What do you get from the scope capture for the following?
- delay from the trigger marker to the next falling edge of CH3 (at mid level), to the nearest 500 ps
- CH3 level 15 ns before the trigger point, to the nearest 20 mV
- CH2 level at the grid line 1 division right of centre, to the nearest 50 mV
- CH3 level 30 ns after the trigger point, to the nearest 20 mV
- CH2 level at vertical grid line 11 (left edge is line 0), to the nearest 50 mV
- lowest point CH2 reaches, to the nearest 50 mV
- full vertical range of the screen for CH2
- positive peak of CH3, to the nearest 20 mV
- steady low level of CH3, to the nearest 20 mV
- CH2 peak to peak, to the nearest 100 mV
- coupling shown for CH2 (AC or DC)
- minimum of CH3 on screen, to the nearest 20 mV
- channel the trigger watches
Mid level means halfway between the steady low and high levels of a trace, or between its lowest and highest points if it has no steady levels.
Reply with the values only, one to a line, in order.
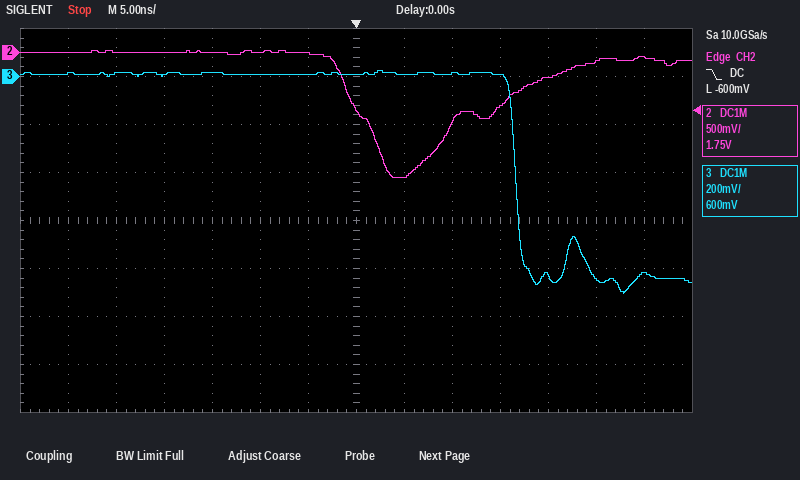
16.5 ns
20 mV
-1.30 V
-820 mV
-250 mV
-1.30 V
4 V
20 mV
-840 mV
1.30 V
DC
-900 mV
CH2
